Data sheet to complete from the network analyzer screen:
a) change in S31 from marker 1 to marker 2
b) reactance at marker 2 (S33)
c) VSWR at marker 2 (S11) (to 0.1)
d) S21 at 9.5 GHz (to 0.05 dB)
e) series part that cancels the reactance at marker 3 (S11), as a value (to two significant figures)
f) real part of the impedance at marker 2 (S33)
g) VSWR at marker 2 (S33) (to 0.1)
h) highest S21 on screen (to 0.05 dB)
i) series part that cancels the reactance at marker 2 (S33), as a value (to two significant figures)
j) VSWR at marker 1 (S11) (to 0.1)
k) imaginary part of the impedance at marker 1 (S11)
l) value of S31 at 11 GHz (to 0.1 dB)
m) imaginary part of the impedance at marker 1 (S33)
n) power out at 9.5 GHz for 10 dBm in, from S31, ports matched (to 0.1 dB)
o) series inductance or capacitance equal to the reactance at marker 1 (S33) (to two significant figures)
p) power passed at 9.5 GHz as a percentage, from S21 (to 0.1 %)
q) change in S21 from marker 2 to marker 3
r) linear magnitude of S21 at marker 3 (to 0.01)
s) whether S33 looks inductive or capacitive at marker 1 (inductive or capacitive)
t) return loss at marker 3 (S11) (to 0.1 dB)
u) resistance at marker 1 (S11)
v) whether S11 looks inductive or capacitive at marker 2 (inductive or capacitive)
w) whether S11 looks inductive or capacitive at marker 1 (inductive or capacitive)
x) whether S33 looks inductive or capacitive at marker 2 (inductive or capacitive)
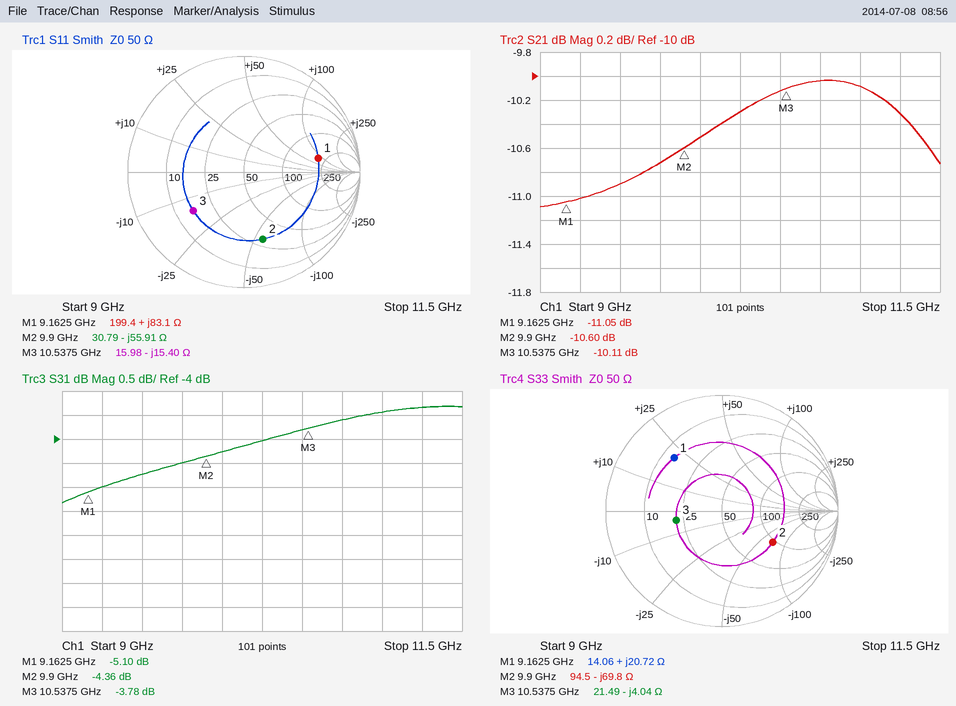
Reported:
0.74 dB
-69.8 Ω
4.0
-10.90 dB
230 pH
94.5 Ω
3.1
-10.05 dB
1.1 nH
4.7
+83.1 Ω
-3.4 dB
+20.72 Ω
5.3 dBm
360 pH
8.1 %
0.49 dB
0.31
inductive
5.2 dB
199.4 Ω
capacitive
inductive
capacitive
